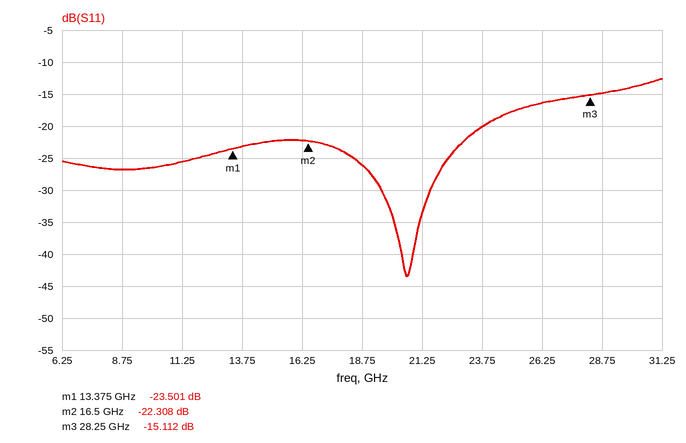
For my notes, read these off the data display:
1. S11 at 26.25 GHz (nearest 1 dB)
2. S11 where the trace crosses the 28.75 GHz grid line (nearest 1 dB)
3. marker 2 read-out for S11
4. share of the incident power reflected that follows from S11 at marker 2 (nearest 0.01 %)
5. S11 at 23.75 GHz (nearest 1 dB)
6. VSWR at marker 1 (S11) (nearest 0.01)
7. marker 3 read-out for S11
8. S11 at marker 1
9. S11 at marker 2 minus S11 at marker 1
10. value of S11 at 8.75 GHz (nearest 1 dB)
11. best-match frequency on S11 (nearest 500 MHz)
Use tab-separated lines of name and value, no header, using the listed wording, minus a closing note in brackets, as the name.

S11 at 26.25 GHz	-16 dB
S11 where the trace crosses the 28.75 GHz grid line	-15 dB
marker 2 read-out for S11	-22.308 dB
share of the incident power reflected that follows from S11 at marker 2	0.59 %
S11 at 23.75 GHz	-20 dB
VSWR at marker 1 (S11)	1.14
marker 3 read-out for S11	-15.112 dB
S11 at marker 1	-23.501 dB
S11 at marker 2 minus S11 at marker 1	1.193 dB
value of S11 at 8.75 GHz	-27 dB
best-match frequency on S11	20.5 GHz
